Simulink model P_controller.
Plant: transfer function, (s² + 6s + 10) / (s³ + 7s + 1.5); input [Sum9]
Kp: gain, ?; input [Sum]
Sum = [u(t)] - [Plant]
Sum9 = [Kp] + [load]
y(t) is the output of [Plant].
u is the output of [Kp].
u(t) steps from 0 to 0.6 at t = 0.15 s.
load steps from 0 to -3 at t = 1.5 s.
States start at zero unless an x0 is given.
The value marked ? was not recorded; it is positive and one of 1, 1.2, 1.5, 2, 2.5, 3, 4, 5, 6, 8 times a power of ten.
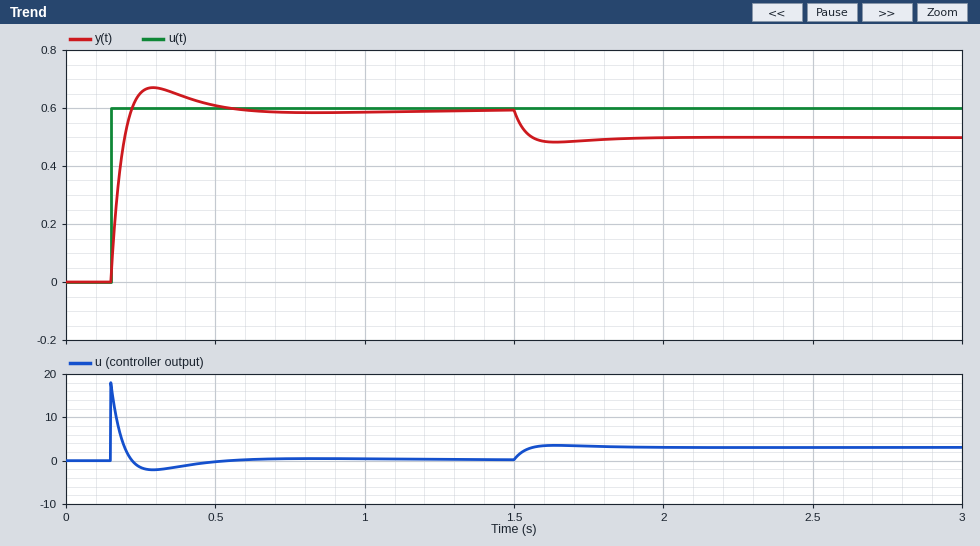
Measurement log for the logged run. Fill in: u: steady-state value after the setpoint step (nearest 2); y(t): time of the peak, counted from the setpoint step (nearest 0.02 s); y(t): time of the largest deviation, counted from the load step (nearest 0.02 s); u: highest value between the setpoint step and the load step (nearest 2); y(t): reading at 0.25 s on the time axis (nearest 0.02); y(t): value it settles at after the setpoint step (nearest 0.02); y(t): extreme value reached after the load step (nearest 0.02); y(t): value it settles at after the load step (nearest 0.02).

0
0.14 s
0.14 s
18
0.66
0.60
0.48
0.50
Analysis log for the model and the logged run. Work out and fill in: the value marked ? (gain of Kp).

30
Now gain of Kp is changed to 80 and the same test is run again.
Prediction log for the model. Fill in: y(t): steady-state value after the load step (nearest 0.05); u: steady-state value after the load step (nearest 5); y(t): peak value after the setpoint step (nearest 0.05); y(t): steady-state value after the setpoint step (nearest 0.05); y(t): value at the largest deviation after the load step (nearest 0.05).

0.55
5
0.65
0.60
0.55
